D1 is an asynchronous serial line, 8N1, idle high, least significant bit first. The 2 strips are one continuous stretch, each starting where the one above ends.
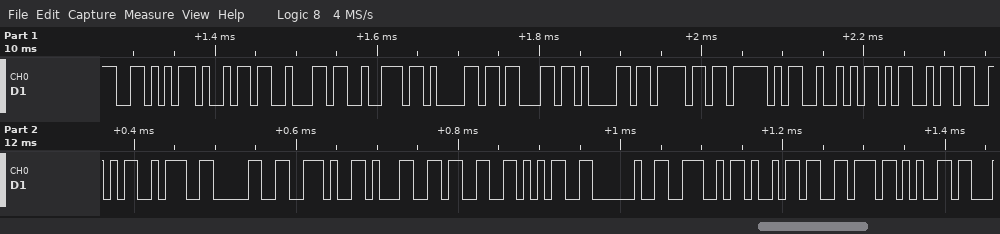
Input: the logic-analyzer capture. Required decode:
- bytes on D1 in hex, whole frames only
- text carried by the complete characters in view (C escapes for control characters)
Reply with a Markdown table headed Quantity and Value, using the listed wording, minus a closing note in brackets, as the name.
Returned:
| Quantity | Value |
|---|---|
| bytes on D1 in hex, whole frames only | 56 69 62 72 61 63 61 6F 5F 52 4D 53 3A 30 2E 31 33 35 20 4E 69 76 65 |
| text carried by the complete characters in view | "Vibracao_RMS:0.135 Nive" |
